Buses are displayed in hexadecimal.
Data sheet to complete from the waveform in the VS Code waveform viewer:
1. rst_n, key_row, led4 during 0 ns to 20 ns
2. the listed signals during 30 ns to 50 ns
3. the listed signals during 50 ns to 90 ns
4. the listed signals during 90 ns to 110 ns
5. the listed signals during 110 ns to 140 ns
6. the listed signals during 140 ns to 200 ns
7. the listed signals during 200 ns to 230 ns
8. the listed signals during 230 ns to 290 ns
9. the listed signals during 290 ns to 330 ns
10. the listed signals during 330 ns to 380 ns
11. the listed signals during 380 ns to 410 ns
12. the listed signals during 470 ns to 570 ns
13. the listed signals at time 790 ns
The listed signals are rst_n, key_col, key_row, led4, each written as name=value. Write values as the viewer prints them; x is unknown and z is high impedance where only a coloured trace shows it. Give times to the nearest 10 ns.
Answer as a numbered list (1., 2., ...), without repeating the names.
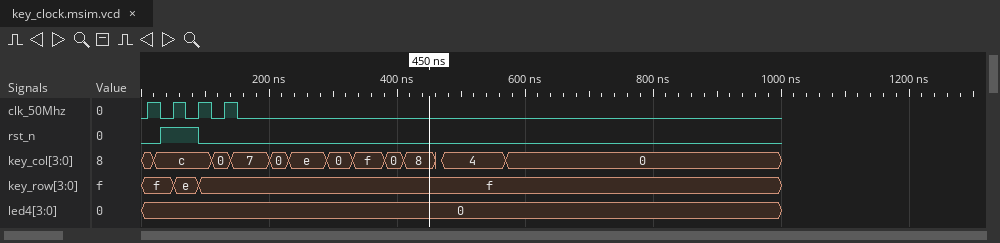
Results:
1. rst_n=0, key_row=f, led4=0
2. rst_n=1, key_col=c, key_row=f, led4=0
3. rst_n=1, key_col=c, key_row=e, led4=0
4. rst_n=0, key_col=c, key_row=f, led4=0
5. rst_n=0, key_col=0, key_row=f, led4=0
6. rst_n=0, key_col=7, key_row=f, led4=0
7. rst_n=0, key_col=0, key_row=f, led4=0
8. rst_n=0, key_col=e, key_row=f, led4=0
9. rst_n=0, key_col=0, key_row=f, led4=0
10. rst_n=0, key_col=f, key_row=f, led4=0
11. rst_n=0, key_col=0, key_row=f, led4=0
12. rst_n=0, key_col=4, key_row=f, led4=0
13. rst_n=0, key_col=0, key_row=f, led4=0
